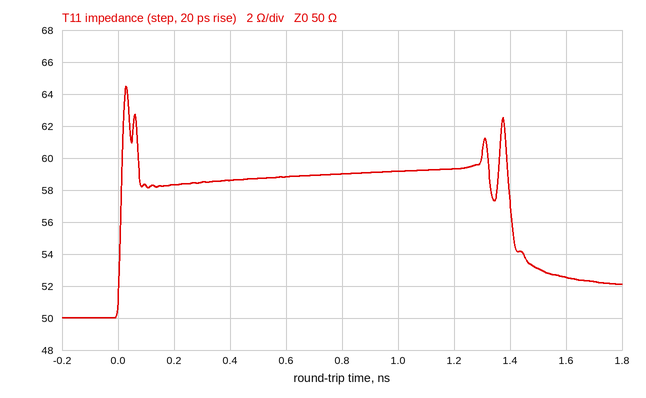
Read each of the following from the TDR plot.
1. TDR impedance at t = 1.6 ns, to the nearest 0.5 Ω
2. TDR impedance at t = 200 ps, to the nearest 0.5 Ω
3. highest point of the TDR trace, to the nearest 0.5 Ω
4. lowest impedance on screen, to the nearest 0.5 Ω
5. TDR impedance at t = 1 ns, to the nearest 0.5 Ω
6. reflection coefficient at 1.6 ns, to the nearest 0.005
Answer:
52.5 Ω
58.5 Ω
64.5 Ω
50.0 Ω
59.0 Ω
+0.025
